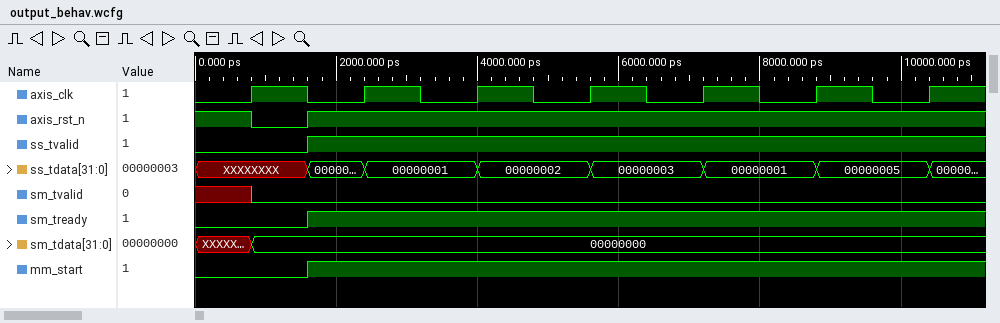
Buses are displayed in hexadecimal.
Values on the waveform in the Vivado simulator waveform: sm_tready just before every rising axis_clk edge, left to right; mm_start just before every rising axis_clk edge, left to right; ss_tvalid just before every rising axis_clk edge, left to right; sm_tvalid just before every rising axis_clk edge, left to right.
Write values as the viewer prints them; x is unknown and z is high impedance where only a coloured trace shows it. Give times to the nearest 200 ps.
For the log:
0 1 1 1 1 1 1
0 1 1 1 1 1 1
0 1 1 1 1 1 1
x 0 0 0 0 0 0
